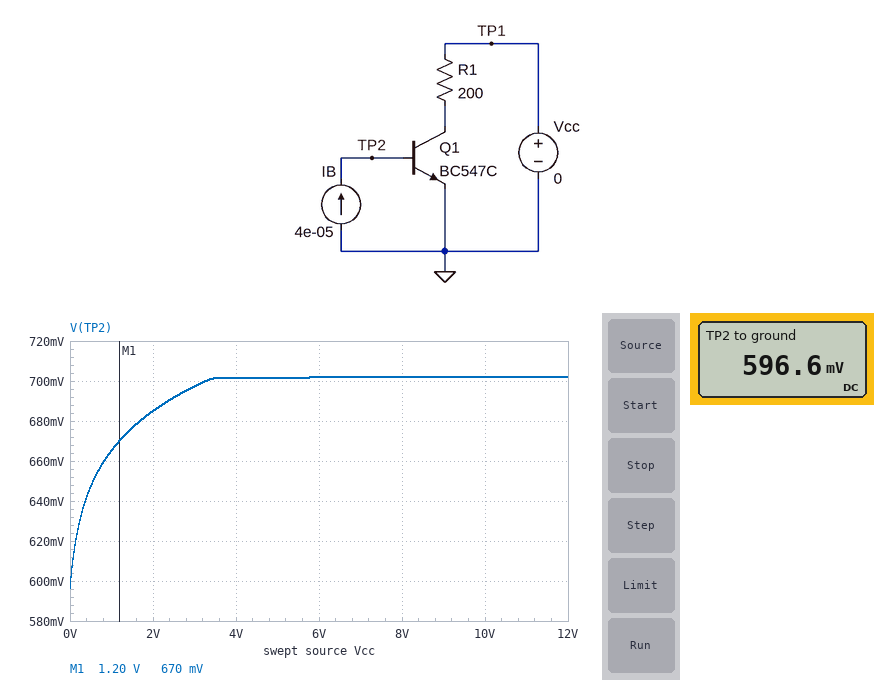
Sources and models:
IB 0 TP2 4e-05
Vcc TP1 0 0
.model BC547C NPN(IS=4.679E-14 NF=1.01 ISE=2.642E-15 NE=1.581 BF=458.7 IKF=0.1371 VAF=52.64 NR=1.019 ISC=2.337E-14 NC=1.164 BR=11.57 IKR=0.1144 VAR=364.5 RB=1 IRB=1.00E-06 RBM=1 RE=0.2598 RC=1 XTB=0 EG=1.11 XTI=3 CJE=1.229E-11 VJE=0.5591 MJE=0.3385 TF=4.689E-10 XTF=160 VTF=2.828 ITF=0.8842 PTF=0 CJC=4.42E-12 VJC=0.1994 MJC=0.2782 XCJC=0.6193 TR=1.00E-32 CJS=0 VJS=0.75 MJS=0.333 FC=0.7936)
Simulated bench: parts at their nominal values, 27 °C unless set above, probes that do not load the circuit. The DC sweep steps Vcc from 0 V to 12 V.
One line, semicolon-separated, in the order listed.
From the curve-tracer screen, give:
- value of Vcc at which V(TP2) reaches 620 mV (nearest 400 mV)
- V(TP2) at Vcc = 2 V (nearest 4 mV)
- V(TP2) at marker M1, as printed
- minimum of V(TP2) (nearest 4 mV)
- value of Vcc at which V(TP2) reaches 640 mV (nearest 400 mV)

0 V; 684 mV; 670 mV; 596 mV; 400 mV
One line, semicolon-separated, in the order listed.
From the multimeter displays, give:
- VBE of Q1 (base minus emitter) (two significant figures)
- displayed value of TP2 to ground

600 mV; 596.6 mV
